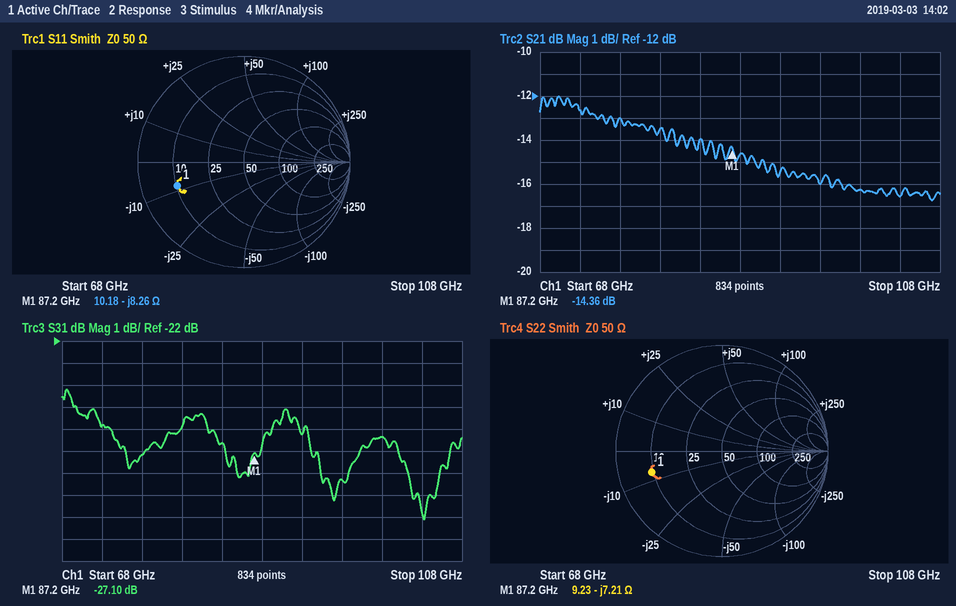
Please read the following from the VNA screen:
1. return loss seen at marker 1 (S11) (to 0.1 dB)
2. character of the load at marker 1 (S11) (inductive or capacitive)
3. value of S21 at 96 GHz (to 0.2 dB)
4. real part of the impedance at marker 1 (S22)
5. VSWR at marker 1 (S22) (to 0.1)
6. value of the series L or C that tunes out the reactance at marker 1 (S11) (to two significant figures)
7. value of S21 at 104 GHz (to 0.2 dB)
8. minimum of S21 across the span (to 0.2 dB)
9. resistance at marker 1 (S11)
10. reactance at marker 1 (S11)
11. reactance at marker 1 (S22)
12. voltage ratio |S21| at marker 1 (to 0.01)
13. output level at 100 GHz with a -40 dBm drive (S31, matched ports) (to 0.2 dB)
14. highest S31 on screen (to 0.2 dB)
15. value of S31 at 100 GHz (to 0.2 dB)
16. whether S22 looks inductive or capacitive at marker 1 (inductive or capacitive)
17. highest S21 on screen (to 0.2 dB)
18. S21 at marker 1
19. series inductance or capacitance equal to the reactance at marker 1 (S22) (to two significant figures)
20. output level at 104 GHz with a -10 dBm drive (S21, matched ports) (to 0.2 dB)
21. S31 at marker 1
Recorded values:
3.5 dB
capacitive
-16.0 dB
9.23 Ω
5.5
15 pH
-16.6 dB
-16.8 dB
10.18 Ω
-8.26 Ω
-7.21 Ω
0.19
-66.4 dBm
-24.2 dB
-26.4 dB
capacitive
-12.0 dB
-14.36 dB
250 fF
-26.6 dBm
-27.10 dB
